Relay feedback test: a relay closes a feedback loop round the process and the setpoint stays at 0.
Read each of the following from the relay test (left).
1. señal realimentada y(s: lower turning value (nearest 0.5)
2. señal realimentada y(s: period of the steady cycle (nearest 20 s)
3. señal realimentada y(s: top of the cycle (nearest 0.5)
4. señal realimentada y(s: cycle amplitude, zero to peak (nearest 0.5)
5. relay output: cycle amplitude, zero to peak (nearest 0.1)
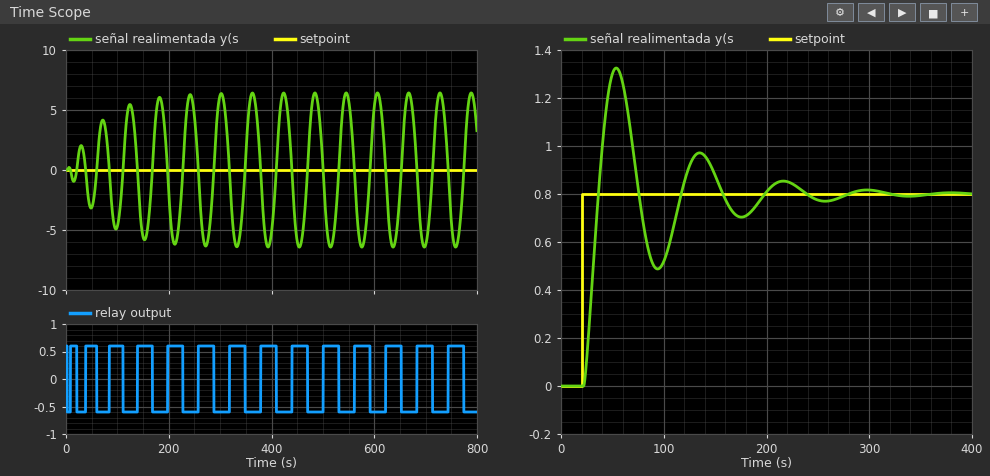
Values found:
-6.5
60 s
6.5
6.5
0.6
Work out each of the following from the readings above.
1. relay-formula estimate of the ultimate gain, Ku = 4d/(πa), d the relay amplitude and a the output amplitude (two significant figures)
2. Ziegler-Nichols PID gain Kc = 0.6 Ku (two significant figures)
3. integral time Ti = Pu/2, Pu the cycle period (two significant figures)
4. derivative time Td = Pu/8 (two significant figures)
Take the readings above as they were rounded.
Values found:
0.12
0.072
30 s
7.5 s
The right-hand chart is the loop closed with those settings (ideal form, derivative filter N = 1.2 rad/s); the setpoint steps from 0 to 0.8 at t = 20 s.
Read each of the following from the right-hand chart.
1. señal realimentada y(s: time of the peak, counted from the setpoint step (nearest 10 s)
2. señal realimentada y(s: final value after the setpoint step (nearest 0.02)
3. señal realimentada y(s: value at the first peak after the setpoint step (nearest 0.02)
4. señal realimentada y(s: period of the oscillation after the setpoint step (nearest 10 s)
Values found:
30 s
0.80
1.32
80 s
